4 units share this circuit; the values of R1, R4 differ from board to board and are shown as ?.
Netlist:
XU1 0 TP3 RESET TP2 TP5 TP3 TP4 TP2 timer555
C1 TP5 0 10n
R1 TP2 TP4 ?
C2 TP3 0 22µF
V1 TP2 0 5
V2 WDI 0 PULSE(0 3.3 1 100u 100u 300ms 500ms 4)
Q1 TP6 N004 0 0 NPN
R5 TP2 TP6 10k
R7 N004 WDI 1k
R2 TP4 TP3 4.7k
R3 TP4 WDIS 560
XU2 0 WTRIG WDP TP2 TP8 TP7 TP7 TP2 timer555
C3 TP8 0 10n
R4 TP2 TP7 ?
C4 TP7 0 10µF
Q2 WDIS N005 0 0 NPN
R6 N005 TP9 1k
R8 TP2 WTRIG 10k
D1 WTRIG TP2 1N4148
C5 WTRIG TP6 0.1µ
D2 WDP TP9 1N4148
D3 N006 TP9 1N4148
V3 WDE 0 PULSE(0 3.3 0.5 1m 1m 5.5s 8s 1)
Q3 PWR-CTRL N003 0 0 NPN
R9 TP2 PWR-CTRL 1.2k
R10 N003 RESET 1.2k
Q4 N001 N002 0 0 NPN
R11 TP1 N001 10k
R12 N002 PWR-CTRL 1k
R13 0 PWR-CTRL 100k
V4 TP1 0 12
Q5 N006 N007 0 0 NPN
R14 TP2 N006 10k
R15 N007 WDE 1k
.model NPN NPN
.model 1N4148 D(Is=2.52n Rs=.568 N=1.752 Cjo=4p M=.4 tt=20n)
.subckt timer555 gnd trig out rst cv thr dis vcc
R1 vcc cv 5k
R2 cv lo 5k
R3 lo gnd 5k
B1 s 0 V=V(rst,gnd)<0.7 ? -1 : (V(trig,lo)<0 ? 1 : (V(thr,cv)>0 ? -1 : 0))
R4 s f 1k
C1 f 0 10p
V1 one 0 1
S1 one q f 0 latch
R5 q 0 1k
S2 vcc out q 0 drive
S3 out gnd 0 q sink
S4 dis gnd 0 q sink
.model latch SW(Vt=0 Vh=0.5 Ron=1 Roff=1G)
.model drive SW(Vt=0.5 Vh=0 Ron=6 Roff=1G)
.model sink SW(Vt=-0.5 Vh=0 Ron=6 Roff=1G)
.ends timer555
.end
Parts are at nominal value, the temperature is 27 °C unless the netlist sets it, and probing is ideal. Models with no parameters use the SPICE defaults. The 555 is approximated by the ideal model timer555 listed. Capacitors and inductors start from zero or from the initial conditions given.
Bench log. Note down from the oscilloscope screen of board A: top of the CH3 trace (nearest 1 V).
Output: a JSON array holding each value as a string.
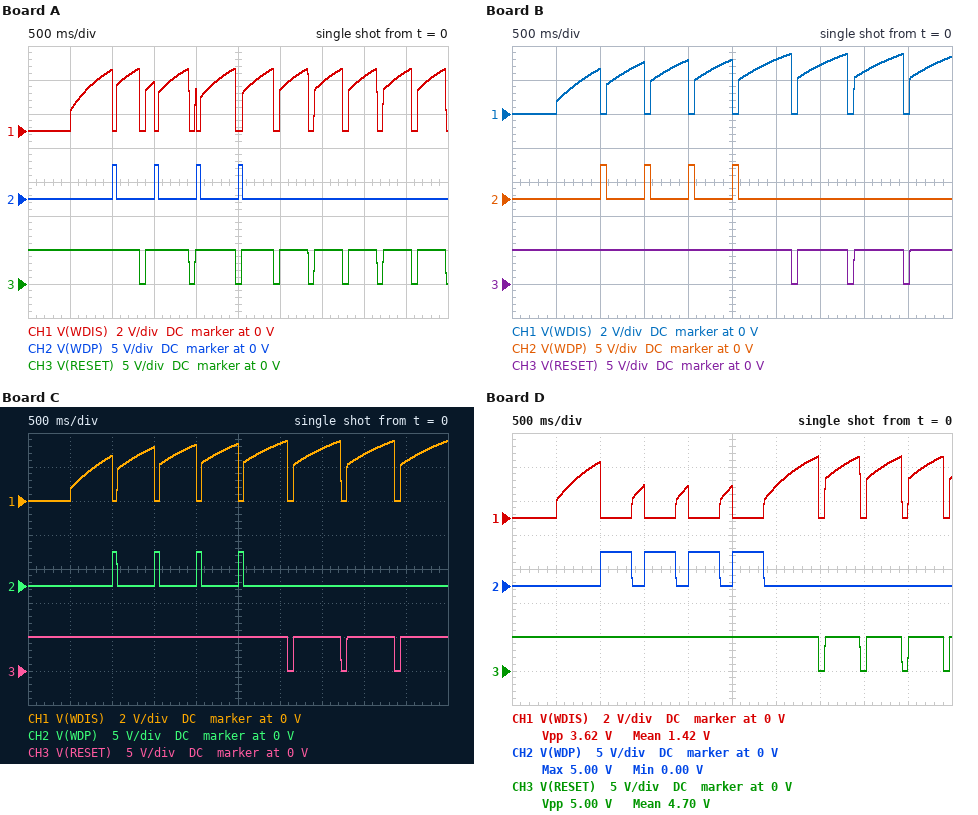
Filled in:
["5 V"]
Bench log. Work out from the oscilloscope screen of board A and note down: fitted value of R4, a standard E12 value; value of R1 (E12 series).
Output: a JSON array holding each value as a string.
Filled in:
["4.7 kΩ", "18 kΩ"]
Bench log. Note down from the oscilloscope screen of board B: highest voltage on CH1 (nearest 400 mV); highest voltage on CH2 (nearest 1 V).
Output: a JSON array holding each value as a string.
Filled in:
["3.6 V", "5 V"]
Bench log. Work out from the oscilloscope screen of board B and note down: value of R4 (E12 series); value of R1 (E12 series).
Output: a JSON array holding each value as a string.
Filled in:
["6.8 kΩ", "33 kΩ"]
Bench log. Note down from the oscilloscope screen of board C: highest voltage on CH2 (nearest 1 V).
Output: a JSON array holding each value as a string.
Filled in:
["5 V"]
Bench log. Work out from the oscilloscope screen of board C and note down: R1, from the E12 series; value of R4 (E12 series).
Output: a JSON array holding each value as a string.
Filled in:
["33 kΩ", "5.6 kΩ"]
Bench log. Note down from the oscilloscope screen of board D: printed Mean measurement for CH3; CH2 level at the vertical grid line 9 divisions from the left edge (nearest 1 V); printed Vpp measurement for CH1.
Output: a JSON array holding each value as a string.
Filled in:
["4.70 V", "0 V", "3.62 V"]
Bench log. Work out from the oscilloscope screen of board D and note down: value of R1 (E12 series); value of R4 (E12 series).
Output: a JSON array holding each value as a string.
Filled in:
["22 kΩ", "33 kΩ"]
